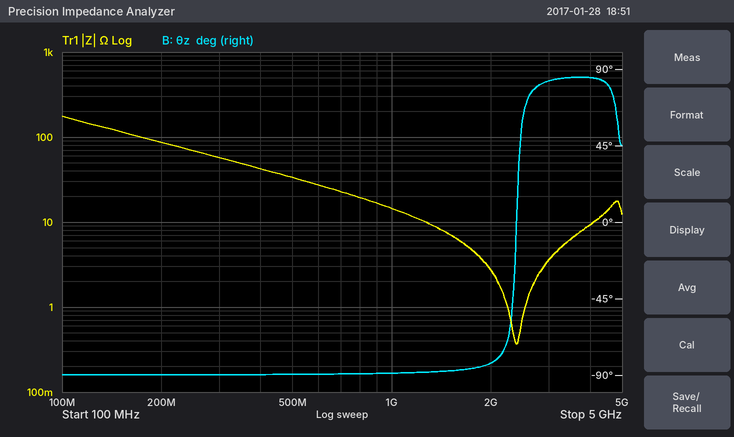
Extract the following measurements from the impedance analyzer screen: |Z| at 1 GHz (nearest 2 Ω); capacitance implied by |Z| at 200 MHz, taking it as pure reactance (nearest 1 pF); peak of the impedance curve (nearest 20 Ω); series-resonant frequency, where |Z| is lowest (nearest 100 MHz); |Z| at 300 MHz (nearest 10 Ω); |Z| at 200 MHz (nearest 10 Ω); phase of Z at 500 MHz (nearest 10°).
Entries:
14 Ω
9 pF
180 Ω
2.4 GHz
60 Ω
90 Ω
-90°
